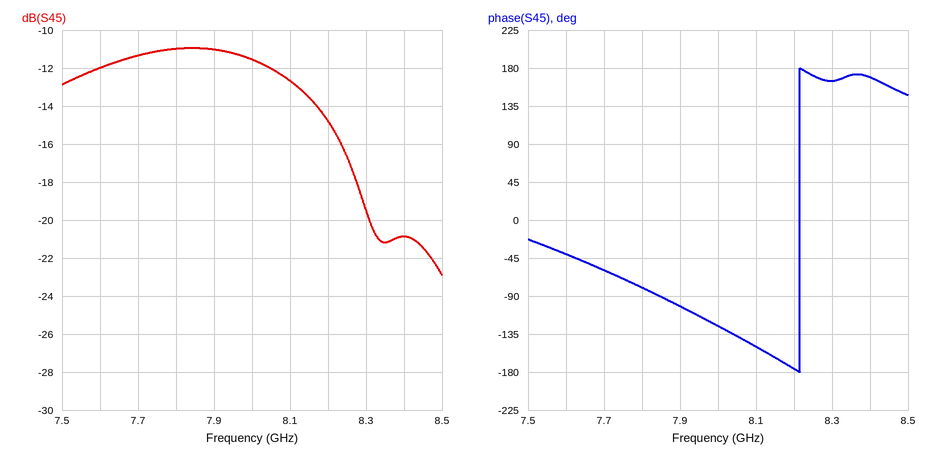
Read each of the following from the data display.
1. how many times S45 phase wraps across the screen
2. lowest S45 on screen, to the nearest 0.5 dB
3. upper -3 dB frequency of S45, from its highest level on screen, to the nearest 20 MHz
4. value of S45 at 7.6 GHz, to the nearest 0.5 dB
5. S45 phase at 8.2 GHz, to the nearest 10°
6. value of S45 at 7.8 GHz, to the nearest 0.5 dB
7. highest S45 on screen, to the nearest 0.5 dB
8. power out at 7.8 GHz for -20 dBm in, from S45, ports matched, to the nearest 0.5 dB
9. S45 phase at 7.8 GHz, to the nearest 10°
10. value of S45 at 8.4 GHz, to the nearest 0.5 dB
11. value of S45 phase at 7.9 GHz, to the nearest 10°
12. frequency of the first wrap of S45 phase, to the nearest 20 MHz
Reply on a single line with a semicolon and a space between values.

1; -23.0 dB; 8.16 GHz; -12.0 dB; -180°; -11.0 dB; -11.0 dB; -31.0 dBm; -80°; -21.0 dB; -100°; 8.22 GHz
